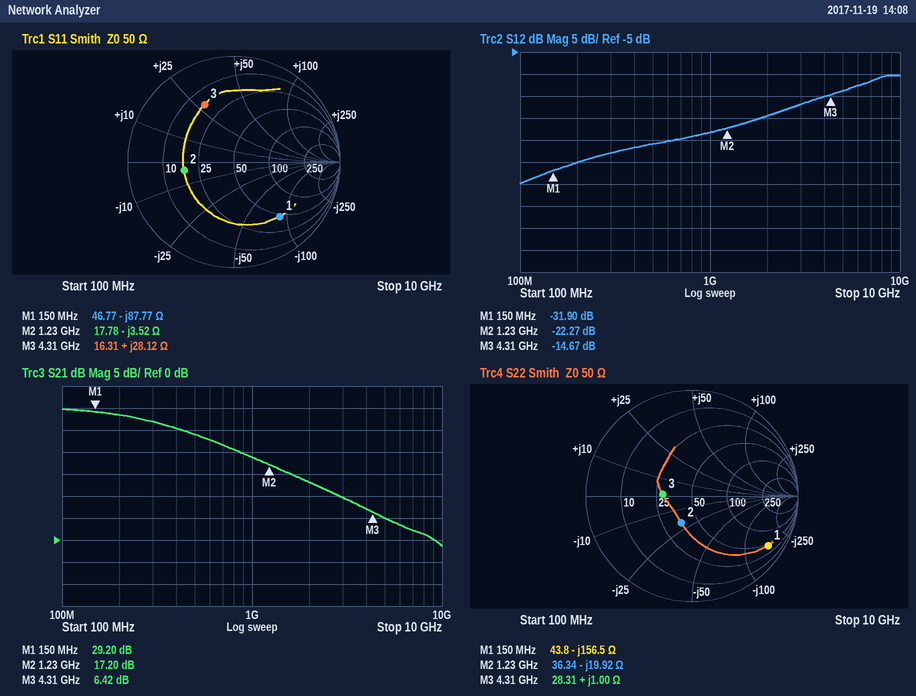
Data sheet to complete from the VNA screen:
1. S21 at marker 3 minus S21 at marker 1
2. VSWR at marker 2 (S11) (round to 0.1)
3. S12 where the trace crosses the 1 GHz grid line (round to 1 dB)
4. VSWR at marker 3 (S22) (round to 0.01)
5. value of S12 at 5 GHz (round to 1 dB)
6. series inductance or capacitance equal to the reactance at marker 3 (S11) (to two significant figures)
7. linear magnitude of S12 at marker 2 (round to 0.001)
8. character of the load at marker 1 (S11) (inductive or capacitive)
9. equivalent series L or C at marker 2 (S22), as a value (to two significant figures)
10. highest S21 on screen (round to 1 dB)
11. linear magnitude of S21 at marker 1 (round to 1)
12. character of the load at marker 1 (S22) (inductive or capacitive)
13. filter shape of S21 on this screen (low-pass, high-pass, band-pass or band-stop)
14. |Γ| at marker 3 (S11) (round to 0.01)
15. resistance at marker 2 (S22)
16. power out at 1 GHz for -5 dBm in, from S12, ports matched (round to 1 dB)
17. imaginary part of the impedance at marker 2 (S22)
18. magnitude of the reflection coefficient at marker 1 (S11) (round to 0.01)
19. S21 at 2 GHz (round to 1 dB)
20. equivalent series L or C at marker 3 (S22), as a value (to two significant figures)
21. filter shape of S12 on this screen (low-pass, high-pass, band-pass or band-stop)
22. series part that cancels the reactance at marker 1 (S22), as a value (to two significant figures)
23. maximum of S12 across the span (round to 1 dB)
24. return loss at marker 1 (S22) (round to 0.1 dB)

-22.78 dB
2.8
-23 dB
1.77
-14 dB
1.0 nH
0.077
capacitive
6.5 pF
30 dB
29
capacitive
low-pass
0.61
36.34 Ω
-28 dBm
-19.92 Ω
0.67
13 dB
37 pH
high-pass
170 nH
-10 dB
1.3 dB
